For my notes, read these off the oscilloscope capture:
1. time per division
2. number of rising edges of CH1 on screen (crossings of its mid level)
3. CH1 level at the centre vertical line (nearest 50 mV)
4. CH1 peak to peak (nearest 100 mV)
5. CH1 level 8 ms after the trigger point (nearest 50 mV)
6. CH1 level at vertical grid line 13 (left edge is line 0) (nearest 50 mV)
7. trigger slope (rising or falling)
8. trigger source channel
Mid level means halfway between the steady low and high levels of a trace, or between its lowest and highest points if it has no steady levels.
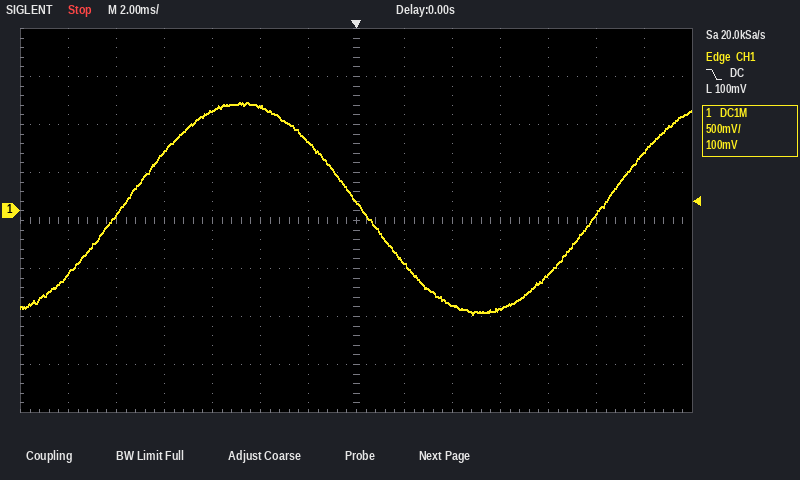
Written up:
2 ms
2
100 mV
2.20 V
-650 mV
600 mV
falling
CH1
